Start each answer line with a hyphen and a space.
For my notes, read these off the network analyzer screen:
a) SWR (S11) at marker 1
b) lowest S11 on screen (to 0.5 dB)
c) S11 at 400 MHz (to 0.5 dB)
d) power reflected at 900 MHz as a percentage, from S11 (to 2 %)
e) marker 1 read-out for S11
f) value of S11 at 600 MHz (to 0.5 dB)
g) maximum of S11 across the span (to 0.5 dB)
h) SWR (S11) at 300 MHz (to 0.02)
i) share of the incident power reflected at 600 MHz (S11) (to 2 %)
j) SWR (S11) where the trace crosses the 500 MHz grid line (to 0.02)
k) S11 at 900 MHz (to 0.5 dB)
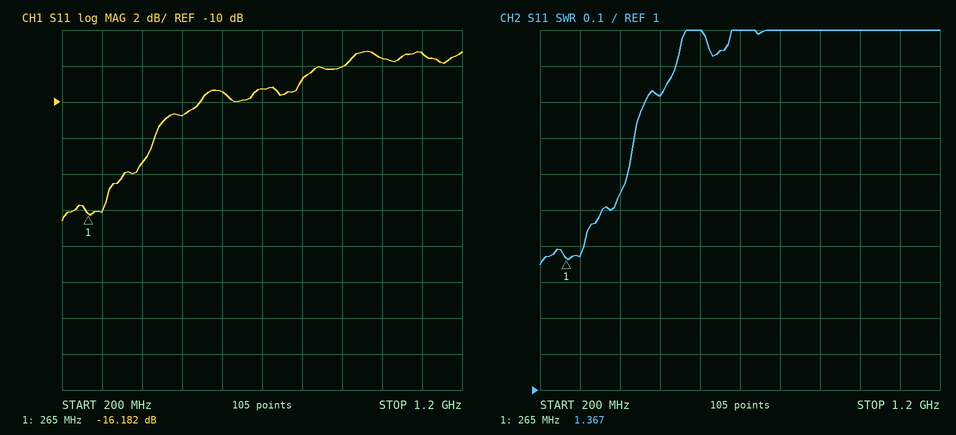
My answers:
- 1.367
- -16.5 dB
- -13.5 dB
- 16 %
- -16.182 dB
- -9.5 dB
- -7.0 dB
- 1.38
- 12 %
- 1.82
- -8.0 dB
